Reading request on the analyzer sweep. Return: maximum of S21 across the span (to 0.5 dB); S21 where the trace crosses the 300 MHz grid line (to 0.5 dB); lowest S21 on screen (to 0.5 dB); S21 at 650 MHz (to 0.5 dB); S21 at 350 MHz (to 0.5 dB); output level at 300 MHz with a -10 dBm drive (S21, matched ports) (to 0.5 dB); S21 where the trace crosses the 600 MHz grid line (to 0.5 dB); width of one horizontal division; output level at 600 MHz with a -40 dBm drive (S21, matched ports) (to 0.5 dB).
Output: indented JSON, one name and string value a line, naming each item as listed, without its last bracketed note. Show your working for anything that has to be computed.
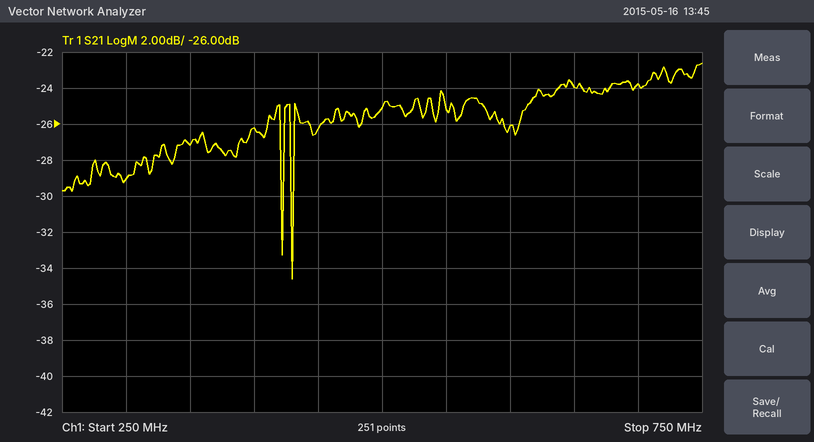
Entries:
{
  "maximum of S21 across the span": "-22.5 dB",
  "S21 where the trace crosses the 300 MHz grid line": "-29.0 dB",
  "lowest S21 on screen": "-34.5 dB",
  "S21 at 650 MHz": "-24.0 dB",
  "S21 at 350 MHz": "-27.0 dB",
  "output level at 300 MHz with a -10 dBm drive (S21, matched ports)": "-10 dBm + (-29.0 dB) = -39.0 dBm",
  "S21 where the trace crosses the 600 MHz grid line": "-26.0 dB",
  "width of one horizontal division": "50 MHz",
  "output level at 600 MHz with a -40 dBm drive (S21, matched ports)": "-40 dBm + (-26.0 dB) = -66.0 dBm"
}
